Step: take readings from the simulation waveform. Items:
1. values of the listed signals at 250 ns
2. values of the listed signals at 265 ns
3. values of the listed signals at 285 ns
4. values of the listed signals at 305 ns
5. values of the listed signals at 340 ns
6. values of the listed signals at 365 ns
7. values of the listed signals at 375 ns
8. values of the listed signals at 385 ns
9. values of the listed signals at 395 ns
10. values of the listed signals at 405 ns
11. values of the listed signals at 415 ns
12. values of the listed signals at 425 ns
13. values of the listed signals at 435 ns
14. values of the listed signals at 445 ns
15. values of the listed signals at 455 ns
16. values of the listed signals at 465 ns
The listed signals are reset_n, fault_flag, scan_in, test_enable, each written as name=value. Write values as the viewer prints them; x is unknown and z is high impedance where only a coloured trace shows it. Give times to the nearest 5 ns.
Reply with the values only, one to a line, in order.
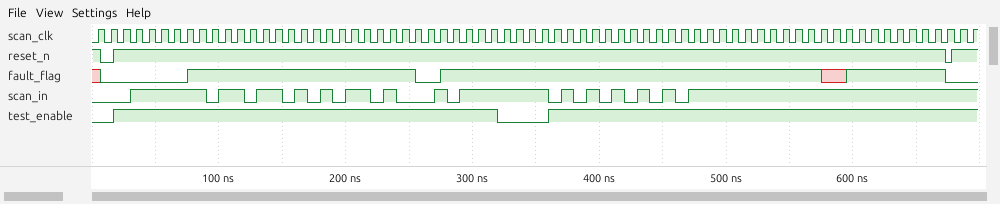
reset_n=1, fault_flag=1, scan_in=0, test_enable=1
reset_n=1, fault_flag=0, scan_in=0, test_enable=1
reset_n=1, fault_flag=1, scan_in=0, test_enable=1
reset_n=1, fault_flag=1, scan_in=1, test_enable=1
reset_n=1, fault_flag=1, scan_in=1, test_enable=0
reset_n=1, fault_flag=1, scan_in=0, test_enable=1
reset_n=1, fault_flag=1, scan_in=1, test_enable=1
reset_n=1, fault_flag=1, scan_in=0, test_enable=1
reset_n=1, fault_flag=1, scan_in=1, test_enable=1
reset_n=1, fault_flag=1, scan_in=0, test_enable=1
reset_n=1, fault_flag=1, scan_in=1, test_enable=1
reset_n=1, fault_flag=1, scan_in=0, test_enable=1
reset_n=1, fault_flag=1, scan_in=1, test_enable=1
reset_n=1, fault_flag=1, scan_in=0, test_enable=1
reset_n=1, fault_flag=1, scan_in=1, test_enable=1
reset_n=1, fault_flag=1, scan_in=0, test_enable=1
